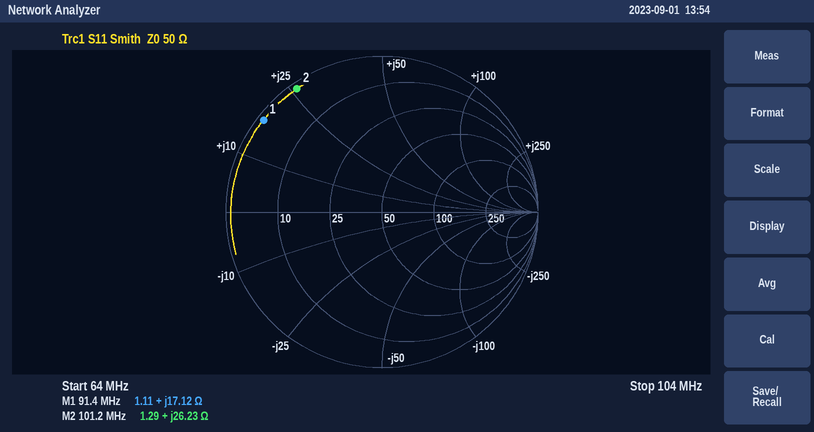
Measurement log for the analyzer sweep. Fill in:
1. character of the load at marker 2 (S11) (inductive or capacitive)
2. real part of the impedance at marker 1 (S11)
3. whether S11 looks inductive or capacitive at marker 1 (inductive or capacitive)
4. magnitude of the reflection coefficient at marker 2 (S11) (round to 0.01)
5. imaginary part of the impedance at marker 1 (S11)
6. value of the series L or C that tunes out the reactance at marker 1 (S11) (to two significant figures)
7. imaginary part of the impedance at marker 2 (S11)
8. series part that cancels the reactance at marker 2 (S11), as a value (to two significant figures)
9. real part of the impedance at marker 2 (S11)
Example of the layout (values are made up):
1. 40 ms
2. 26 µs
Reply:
1. inductive
2. 1.11 Ω
3. inductive
4. 0.96
5. +17.12 Ω
6. 100 pF
7. +26.23 Ω
8. 60 pF
9. 1.29 Ω
